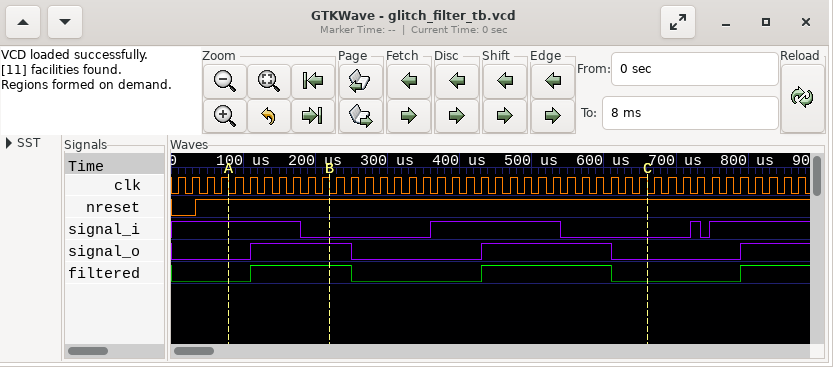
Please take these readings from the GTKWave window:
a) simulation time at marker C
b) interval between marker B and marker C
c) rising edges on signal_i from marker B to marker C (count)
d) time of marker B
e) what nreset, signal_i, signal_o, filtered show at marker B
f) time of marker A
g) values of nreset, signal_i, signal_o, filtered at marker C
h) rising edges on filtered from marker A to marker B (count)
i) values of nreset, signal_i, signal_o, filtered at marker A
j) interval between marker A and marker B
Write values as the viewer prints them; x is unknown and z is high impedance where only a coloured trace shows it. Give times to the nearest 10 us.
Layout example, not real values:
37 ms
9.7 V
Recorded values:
660 us
440 us
1
220 us
nreset=1, signal_i=0, signal_o=1, filtered=1
80 us
nreset=1, signal_i=0, signal_o=0, filtered=0
1
nreset=1, signal_i=1, signal_o=0, filtered=0
140 us
